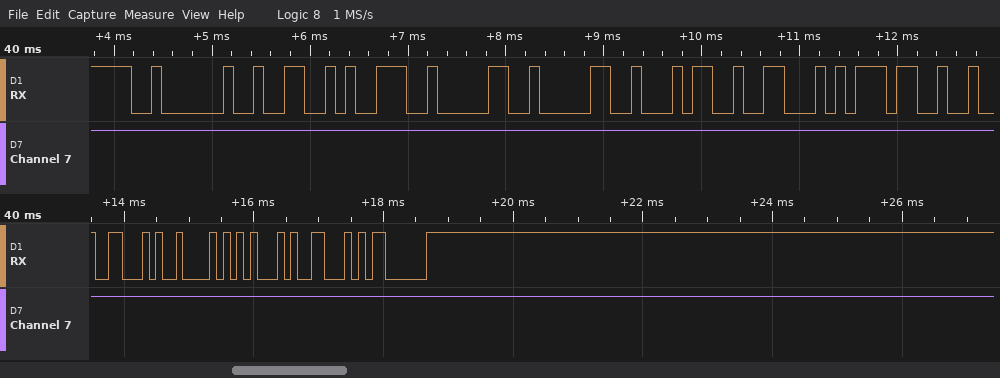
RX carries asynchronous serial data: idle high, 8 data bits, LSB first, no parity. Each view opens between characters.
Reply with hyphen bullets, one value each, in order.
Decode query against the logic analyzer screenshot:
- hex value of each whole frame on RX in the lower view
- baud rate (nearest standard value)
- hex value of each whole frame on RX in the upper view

- 46, 42, 45, 46, 03
- 9600 baud
- 02, 32, 39, 30, 30, 34, 46, 37
